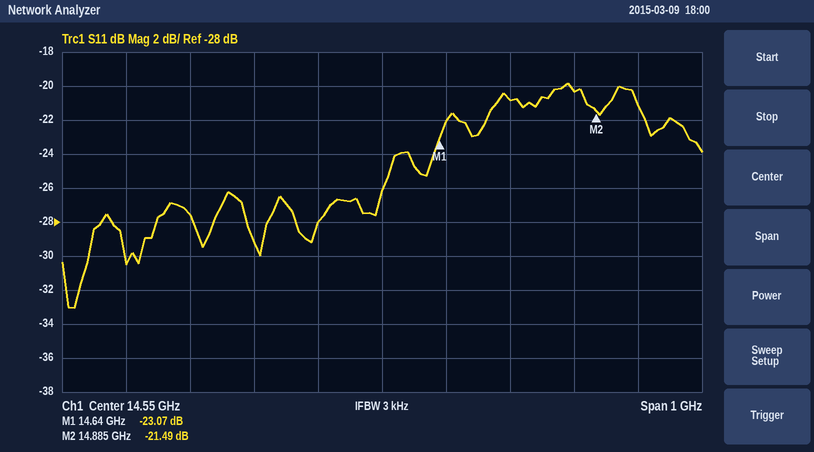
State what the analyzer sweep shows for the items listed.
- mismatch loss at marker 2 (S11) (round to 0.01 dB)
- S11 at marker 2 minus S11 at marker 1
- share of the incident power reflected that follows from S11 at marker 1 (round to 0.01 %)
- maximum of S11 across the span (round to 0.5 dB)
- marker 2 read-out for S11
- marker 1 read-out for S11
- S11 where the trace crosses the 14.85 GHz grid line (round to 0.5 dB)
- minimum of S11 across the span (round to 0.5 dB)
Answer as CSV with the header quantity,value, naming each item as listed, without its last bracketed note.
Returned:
quantity,value
mismatch loss at marker 2 (S11),0.03 dB
S11 at marker 2 minus S11 at marker 1,1.58 dB
share of the incident power reflected that follows from S11 at marker 1,0.49 %
maximum of S11 across the span,-20.0 dB
marker 2 read-out for S11,-21.49 dB
marker 1 read-out for S11,-23.07 dB
S11 where the trace crosses the 14.85 GHz grid line,-20.5 dB
minimum of S11 across the span,-33.0 dB
